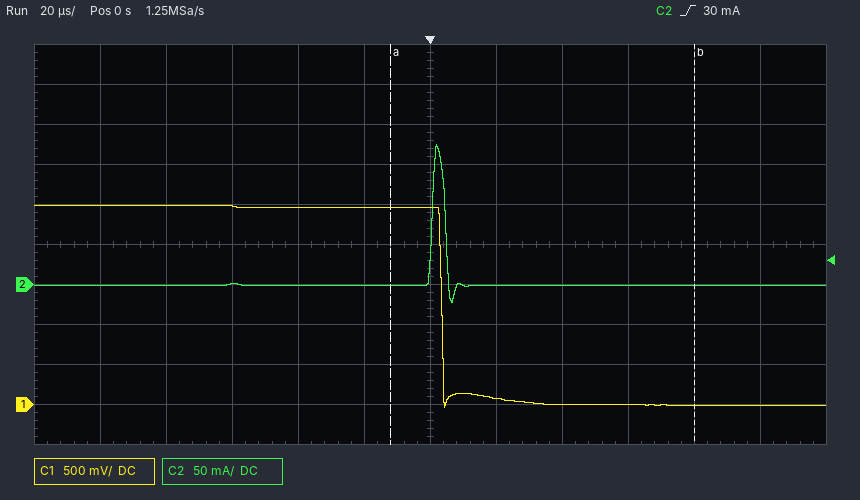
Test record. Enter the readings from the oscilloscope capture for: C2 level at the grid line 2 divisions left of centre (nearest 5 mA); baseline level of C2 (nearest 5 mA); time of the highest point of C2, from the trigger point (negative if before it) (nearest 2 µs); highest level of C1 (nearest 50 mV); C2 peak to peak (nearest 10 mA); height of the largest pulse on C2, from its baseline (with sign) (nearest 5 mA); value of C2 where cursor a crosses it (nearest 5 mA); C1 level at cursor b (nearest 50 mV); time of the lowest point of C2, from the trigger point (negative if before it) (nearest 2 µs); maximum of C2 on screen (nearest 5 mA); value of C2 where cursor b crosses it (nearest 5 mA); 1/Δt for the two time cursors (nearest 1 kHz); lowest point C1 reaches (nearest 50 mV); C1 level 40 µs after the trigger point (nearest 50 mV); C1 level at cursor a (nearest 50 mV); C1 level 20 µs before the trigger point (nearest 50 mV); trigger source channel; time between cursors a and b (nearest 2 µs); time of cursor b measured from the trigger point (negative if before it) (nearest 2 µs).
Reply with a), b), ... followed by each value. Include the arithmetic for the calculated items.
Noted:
a) 0 mA
b) 0 mA
c) +2 µs
d) 2.50 V
e) 200 mA
f) 175 mA − (0 mA) = +175 mA
g) 0 mA
h) 0 mV
i) +6 µs
j) 175 mA
k) 0 mA
l) 1 / 92 µs ≈ 11 kHz
m) -50 mV
n) 0 mV
o) 2.45 V
p) 2.45 V
q) C2
r) 92 µs
s) +80 µs
